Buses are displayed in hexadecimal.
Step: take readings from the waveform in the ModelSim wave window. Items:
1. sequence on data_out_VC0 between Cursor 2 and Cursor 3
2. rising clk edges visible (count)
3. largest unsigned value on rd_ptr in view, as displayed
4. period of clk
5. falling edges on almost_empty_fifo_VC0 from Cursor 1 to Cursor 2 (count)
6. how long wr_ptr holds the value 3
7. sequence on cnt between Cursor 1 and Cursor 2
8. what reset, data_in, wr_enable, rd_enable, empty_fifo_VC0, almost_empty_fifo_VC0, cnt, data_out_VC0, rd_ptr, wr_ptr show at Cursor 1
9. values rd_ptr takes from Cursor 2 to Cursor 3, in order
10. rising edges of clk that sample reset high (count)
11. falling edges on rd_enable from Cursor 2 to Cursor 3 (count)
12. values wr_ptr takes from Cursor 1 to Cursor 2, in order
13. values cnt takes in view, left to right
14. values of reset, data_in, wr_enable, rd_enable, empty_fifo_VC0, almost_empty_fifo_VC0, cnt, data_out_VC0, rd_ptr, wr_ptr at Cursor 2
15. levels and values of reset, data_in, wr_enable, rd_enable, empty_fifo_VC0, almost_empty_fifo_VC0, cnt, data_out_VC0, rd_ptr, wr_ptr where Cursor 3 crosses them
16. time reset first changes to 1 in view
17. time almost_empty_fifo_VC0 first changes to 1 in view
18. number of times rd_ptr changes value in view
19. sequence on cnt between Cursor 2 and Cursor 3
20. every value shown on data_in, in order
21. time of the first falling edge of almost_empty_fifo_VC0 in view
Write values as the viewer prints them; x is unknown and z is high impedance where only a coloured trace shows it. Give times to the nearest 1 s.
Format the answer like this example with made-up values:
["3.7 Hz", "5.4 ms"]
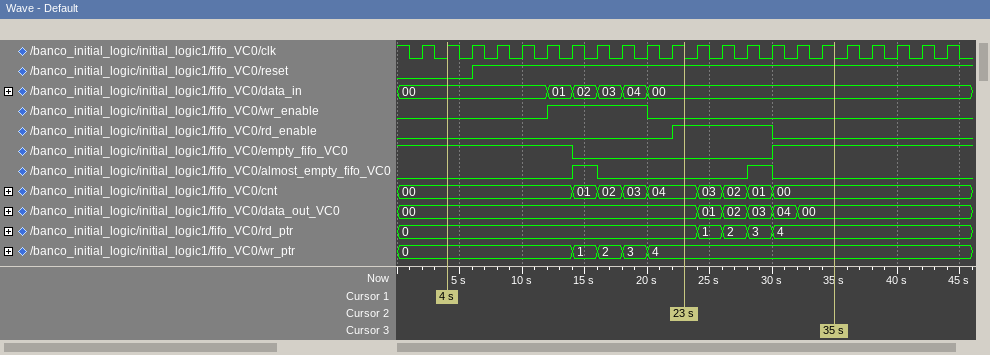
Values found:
["00, 01, 02, 03, 04, 00", "22", "4", "2 s", "1", "2 s", "00, 01, 02, 03, 04", "reset=0, data_in=00, wr_enable=0, rd_enable=0, empty_fifo_VC0=1, almost_empty_fifo_VC0=0, cnt=00, data_out_VC0=00, rd_ptr=0, wr_ptr=0", "0, 1, 2, 3, 4", "19", "1", "0, 1, 2, 3, 4", "00, 01, 02, 03, 04, 03, 02, 01, 00", "reset=1, data_in=00, wr_enable=0, rd_enable=1, empty_fifo_VC0=0, almost_empty_fifo_VC0=0, cnt=04, data_out_VC0=00, rd_ptr=0, wr_ptr=4", "reset=1, data_in=00, wr_enable=0, rd_enable=0, empty_fifo_VC0=1, almost_empty_fifo_VC0=0, cnt=00, data_out_VC0=00, rd_ptr=4, wr_ptr=4", "6 s", "14 s", "4", "04, 03, 02, 01, 00", "00, 01, 02, 03, 04, 00", "16 s"]
